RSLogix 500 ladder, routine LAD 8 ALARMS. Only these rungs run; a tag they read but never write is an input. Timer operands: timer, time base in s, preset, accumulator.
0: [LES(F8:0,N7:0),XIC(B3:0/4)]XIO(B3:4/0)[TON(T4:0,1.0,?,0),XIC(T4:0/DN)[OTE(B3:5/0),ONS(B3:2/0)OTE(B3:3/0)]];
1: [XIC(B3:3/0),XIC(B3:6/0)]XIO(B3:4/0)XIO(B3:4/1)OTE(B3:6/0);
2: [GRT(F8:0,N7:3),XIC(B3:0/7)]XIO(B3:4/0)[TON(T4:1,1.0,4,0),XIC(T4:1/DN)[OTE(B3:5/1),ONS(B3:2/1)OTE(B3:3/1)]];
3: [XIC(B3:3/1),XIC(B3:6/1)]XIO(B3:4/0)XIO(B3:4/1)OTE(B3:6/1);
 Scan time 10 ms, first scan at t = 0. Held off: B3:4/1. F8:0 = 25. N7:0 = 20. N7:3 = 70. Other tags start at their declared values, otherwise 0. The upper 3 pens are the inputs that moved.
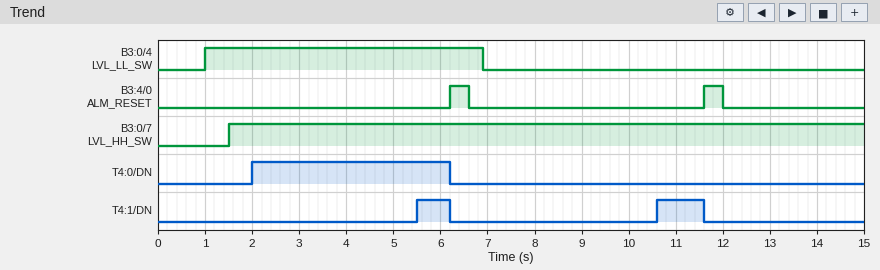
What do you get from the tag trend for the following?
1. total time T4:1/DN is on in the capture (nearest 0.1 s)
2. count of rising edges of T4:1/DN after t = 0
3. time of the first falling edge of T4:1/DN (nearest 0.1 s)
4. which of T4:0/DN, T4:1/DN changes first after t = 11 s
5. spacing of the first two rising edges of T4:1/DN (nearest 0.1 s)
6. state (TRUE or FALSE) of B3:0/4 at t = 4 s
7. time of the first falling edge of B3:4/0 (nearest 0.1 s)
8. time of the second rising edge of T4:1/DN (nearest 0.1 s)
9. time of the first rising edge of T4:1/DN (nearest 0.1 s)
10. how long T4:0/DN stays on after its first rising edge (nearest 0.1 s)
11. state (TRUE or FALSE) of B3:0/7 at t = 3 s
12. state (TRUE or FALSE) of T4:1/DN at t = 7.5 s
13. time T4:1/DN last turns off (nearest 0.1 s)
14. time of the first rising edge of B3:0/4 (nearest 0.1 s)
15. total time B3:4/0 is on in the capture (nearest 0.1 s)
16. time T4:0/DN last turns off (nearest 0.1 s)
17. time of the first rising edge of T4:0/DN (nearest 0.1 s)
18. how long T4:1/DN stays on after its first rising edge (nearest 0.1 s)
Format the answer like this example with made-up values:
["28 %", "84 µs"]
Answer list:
["1.7 s", "2", "6.2 s", "T4:1/DN", "5.1 s", "TRUE", "6.6 s", "10.6 s", "5.5 s", "4.2 s", "TRUE", "FALSE", "11.6 s", "1.0 s", "0.8 s", "6.2 s", "2.0 s", "0.7 s"]
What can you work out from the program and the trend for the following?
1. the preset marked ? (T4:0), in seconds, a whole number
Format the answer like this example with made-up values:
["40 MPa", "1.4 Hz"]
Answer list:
["1 s"]
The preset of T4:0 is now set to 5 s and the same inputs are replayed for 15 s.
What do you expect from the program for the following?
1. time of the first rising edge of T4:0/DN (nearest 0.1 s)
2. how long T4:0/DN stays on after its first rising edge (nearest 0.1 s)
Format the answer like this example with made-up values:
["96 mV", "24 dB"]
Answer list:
["6.0 s", "0.2 s"]
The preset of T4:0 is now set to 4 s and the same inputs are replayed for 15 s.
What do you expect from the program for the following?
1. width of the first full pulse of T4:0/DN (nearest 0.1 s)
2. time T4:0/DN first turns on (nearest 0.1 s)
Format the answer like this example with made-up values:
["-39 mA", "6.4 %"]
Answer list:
["1.2 s", "5.0 s"]
